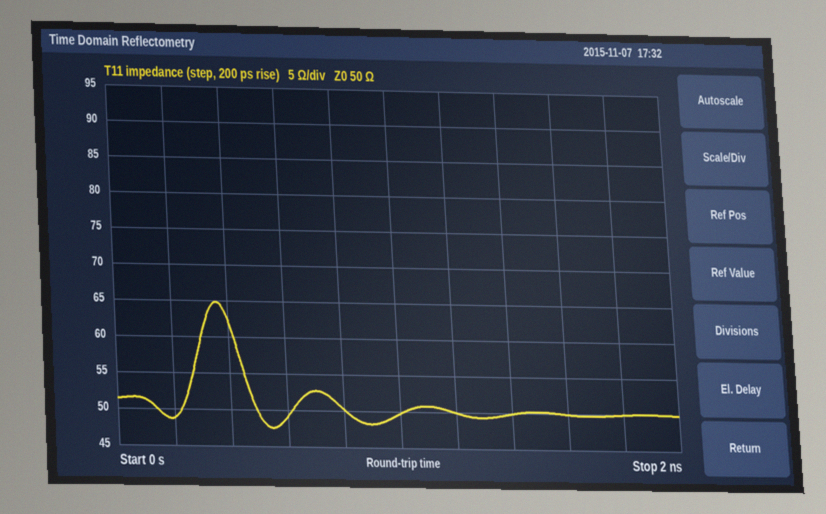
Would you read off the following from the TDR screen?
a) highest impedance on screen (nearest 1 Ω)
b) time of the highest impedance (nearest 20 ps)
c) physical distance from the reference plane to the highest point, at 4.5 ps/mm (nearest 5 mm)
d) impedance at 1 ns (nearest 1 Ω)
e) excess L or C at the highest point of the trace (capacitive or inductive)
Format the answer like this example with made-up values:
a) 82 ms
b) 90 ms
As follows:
a) 65 Ω
b) 360 ps
c) 40 mm
d) 50 Ω
e) inductive
